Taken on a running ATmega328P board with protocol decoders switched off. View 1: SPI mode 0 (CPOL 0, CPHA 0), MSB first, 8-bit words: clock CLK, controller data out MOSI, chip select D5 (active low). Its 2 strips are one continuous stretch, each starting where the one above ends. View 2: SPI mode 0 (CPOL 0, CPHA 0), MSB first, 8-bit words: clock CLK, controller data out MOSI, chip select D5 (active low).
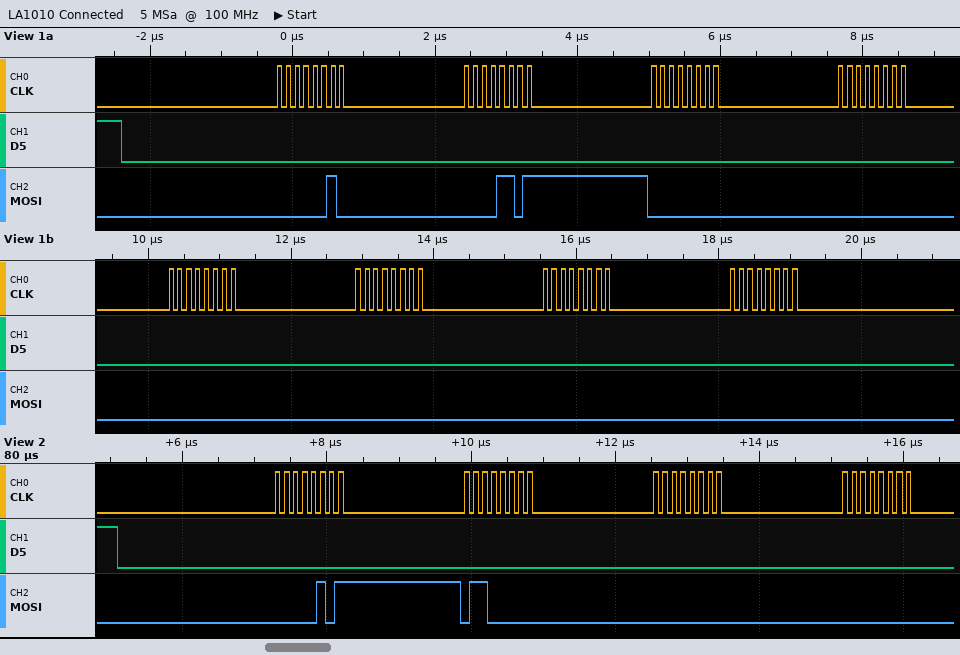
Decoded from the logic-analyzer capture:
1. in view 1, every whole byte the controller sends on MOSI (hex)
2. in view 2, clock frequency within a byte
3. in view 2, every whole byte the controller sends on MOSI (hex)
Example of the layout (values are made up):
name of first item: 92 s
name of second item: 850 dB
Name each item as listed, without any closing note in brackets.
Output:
in view 1, every whole byte the controller sends on MOSI: 02 0D 00 00 00 00 00 00
in view 2, clock frequency within a byte: 8 MHz
in view 2, every whole byte the controller sends on MOSI: 05 60 00 00
